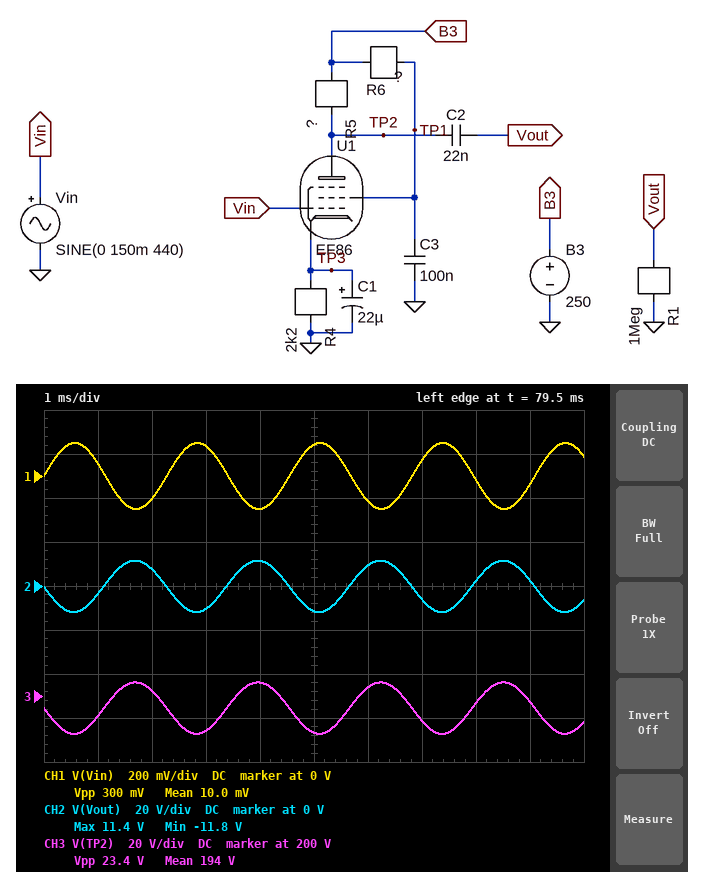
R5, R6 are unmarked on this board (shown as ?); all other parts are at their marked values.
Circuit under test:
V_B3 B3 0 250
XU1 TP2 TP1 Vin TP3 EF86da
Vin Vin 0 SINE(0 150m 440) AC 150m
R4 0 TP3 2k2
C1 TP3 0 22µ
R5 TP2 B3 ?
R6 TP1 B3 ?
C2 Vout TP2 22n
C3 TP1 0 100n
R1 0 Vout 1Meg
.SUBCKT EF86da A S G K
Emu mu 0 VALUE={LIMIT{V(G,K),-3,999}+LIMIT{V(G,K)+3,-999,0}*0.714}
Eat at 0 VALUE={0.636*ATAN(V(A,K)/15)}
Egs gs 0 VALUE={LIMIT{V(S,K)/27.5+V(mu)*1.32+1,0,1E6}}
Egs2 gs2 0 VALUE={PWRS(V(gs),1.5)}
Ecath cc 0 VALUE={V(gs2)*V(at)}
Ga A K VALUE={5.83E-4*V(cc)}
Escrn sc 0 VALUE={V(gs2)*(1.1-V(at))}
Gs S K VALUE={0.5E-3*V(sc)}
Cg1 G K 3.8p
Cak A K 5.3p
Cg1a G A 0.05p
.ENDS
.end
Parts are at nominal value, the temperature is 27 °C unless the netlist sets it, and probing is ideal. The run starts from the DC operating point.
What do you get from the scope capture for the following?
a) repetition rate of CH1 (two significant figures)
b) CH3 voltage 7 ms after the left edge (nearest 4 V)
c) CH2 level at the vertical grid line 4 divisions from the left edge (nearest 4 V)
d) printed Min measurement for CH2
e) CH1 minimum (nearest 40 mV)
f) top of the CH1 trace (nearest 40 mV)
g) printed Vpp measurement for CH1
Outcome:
440 Hz
188 V
12 V
-11.8 V
-160 mV
160 mV
300 mV
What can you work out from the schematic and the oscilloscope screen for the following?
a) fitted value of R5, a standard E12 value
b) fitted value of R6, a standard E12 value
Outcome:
68 kΩ
1.5 MΩ
